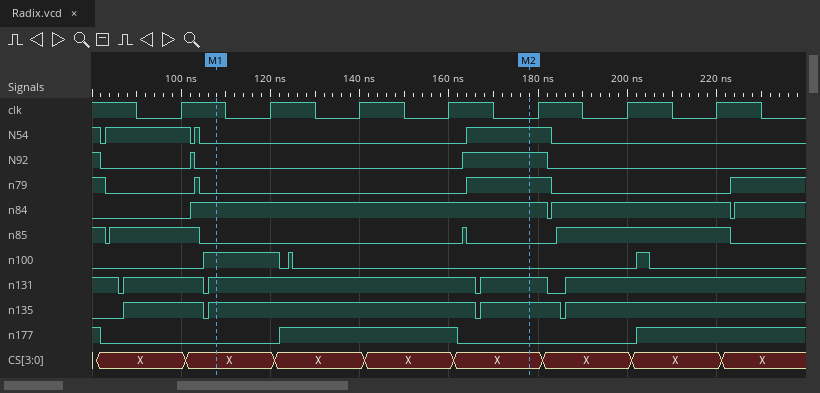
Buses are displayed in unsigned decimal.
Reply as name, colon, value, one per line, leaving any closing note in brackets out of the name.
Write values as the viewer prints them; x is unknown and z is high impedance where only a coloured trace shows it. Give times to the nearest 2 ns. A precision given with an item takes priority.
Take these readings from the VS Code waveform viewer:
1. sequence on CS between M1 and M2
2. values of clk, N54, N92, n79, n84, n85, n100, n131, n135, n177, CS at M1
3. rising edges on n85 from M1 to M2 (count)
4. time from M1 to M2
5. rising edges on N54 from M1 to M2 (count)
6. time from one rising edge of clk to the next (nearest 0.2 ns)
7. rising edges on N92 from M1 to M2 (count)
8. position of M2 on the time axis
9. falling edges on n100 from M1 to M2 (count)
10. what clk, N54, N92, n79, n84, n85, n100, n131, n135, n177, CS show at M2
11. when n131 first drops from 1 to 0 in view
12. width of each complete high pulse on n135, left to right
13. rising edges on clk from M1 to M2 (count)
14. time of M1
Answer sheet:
sequence on CS between M1 and M2: X, X, X, X
values of clk, N54, N92, n79, n84, n85, n100, n131, n135, n177, CS at M1: clk=1, N54=0, N92=0, n79=0, n84=1, n85=0, n100=1, n131=1, n135=1, n177=0, CS=X
rising edges on n85 from M1 to M2: 1
time from M1 to M2: 70 ns
rising edges on N54 from M1 to M2: 1
time from one rising edge of clk to the next: 20 ns
rising edges on N92 from M1 to M2: 1
position of M2 on the time axis: 178 ns
falling edges on n100 from M1 to M2: 2
what clk, N54, N92, n79, n84, n85, n100, n131, n135, n177, CS show at M2: clk=0, N54=1, N92=1, n79=1, n84=1, n85=0, n100=0, n131=1, n135=1, n177=0, CS=X
when n131 first drops from 1 to 0 in view: 86 ns
width of each complete high pulse on n135, left to right: 18 ns, 60 ns, 18 ns
rising edges on clk from M1 to M2: 3
time of M1: 108 ns
